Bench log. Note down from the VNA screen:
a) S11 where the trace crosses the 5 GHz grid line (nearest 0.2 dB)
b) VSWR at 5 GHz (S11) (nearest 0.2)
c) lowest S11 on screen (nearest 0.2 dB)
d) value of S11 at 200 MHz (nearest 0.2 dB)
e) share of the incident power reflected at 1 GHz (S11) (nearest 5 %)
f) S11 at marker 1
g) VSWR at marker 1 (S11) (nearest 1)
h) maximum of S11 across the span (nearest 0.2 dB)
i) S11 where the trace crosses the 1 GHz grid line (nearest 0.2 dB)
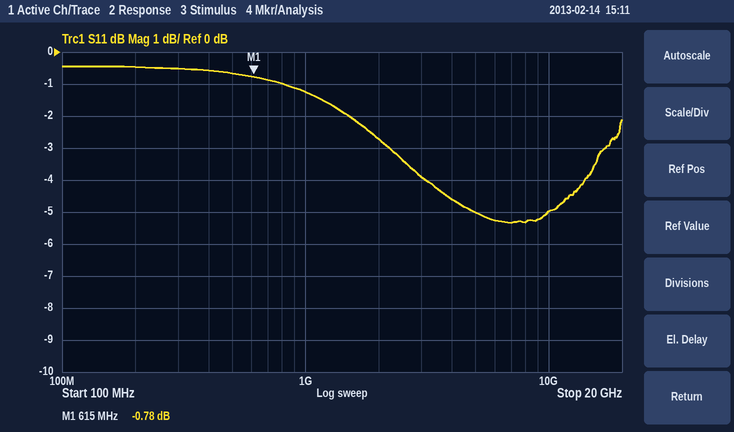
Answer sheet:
-5.0 dB
3.6
-5.4 dB
-0.4 dB
75 %
-0.78 dB
22
-0.4 dB
-1.2 dB
